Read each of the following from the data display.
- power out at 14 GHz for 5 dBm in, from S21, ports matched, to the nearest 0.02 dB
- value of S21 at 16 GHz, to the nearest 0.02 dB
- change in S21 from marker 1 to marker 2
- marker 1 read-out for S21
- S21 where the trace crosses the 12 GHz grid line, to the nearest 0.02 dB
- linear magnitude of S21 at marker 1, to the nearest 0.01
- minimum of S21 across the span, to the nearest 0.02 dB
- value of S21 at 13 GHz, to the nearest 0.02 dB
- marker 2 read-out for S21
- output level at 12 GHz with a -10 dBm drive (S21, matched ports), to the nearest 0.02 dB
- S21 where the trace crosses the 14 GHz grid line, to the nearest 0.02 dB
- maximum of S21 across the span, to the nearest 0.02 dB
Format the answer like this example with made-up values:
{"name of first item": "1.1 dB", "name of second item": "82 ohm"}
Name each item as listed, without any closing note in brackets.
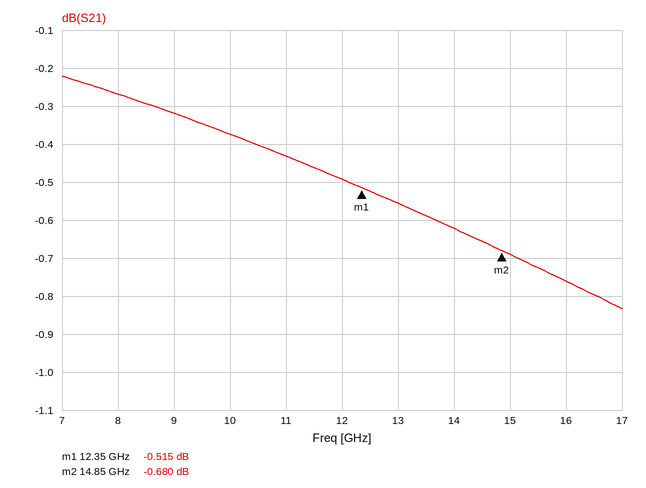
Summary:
{"power out at 14 GHz for 5 dBm in, from S21, ports matched, to the nearest 0.02 dB": "4.38 dBm", "value of S21 at 16 GHz, to the nearest 0.02 dB": "-0.76 dB", "change in S21 from marker 1 to marker 2": "-0.165 dB", "marker 1 read-out for S21": "-0.515 dB", "S21 where the trace crosses the 12 GHz grid line, to the nearest 0.02 dB": "-0.50 dB", "linear magnitude of S21 at marker 1, to the nearest 0.01": "0.94", "minimum of S21 across the span, to the nearest 0.02 dB": "-0.84 dB", "value of S21 at 13 GHz, to the nearest 0.02 dB": "-0.56 dB", "marker 2 read-out for S21": "-0.680 dB", "output level at 12 GHz with a -10 dBm drive (S21, matched ports), to the nearest 0.02 dB": "-10.50 dBm", "S21 where the trace crosses the 14 GHz grid line, to the nearest 0.02 dB": "-0.62 dB", "maximum of S21 across the span, to the nearest 0.02 dB": "-0.22 dB"}
